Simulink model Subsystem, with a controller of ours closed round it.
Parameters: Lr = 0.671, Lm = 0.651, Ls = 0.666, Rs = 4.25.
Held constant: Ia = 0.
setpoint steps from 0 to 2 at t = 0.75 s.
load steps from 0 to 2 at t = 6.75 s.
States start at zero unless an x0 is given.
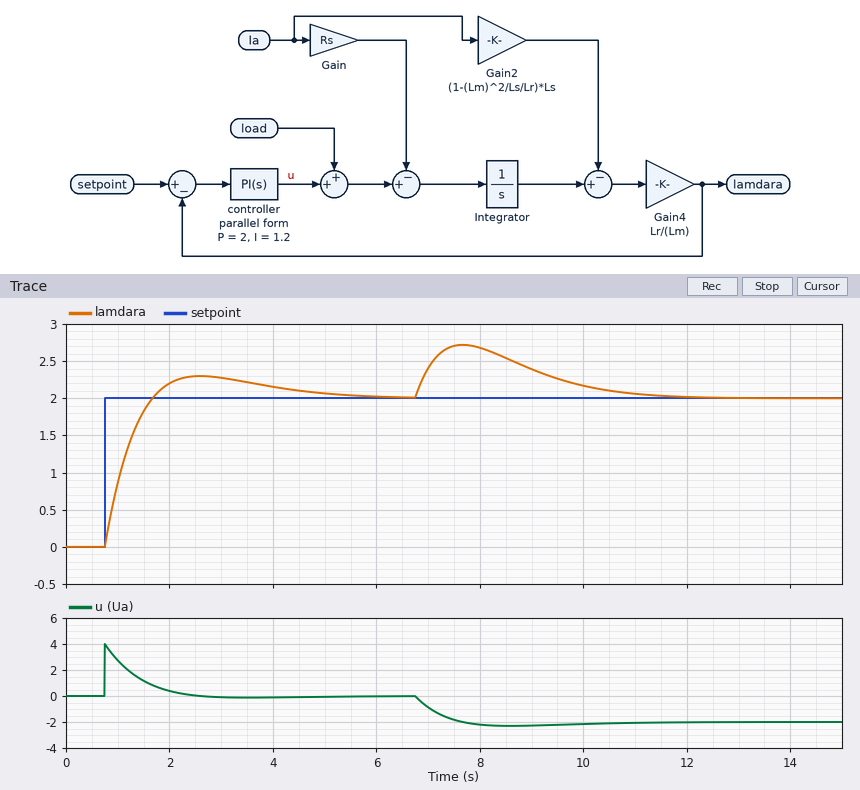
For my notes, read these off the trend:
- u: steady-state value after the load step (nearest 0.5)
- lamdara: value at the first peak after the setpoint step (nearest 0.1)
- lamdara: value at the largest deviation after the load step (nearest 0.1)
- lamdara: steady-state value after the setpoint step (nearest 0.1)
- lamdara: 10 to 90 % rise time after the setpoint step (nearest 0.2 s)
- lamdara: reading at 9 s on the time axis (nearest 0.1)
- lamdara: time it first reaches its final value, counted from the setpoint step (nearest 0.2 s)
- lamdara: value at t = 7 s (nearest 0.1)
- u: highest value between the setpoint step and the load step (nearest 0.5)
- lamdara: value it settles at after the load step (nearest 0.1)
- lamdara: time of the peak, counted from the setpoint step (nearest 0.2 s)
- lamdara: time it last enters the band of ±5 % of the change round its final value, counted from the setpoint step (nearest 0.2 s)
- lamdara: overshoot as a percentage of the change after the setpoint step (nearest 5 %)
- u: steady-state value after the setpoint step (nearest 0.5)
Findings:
-2.0
2.3
2.7
2.0
0.6 s
2.4
1.0 s
2.4
4.0
2.0
1.8 s
3.8 s
15 %
0.0
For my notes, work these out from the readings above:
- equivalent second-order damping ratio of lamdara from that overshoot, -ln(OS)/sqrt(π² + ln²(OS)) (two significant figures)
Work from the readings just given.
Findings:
0.52
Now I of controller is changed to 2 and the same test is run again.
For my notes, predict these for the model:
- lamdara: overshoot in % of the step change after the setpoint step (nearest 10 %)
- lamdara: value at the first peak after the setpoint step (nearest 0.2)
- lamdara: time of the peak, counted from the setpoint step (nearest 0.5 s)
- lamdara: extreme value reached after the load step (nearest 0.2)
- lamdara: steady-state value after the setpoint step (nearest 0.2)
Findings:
20 %
2.4
1.5 s
2.6
2.0
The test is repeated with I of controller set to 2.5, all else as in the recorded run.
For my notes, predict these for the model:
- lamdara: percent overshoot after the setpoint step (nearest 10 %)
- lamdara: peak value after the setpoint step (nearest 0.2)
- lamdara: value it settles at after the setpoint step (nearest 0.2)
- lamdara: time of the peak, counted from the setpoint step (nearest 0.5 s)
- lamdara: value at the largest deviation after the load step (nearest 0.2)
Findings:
20 %
2.4
2.0
1.5 s
2.6
